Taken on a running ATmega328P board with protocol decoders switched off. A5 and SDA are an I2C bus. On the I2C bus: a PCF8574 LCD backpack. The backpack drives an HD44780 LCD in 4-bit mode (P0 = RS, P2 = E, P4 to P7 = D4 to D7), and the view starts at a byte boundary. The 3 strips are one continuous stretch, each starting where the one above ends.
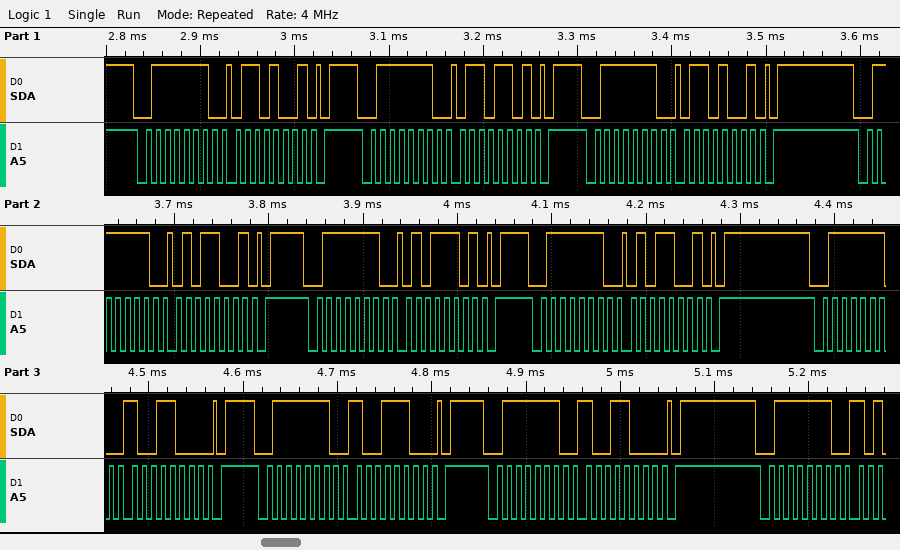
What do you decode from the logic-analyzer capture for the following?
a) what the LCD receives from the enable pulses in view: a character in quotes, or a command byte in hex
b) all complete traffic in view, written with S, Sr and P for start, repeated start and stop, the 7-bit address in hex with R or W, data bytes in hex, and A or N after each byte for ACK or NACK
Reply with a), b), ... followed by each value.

a) 'e'
b) S 3FW A 69 A P S 3FW A 6D A P S 3FW A 69 A P S 3FW A 59 A P S 3FW A 5D A P S 3FW A 59 A P S 3FW A 98 A P S 3FW A 9C A P S 3FW A 98 A P S 3FW A
